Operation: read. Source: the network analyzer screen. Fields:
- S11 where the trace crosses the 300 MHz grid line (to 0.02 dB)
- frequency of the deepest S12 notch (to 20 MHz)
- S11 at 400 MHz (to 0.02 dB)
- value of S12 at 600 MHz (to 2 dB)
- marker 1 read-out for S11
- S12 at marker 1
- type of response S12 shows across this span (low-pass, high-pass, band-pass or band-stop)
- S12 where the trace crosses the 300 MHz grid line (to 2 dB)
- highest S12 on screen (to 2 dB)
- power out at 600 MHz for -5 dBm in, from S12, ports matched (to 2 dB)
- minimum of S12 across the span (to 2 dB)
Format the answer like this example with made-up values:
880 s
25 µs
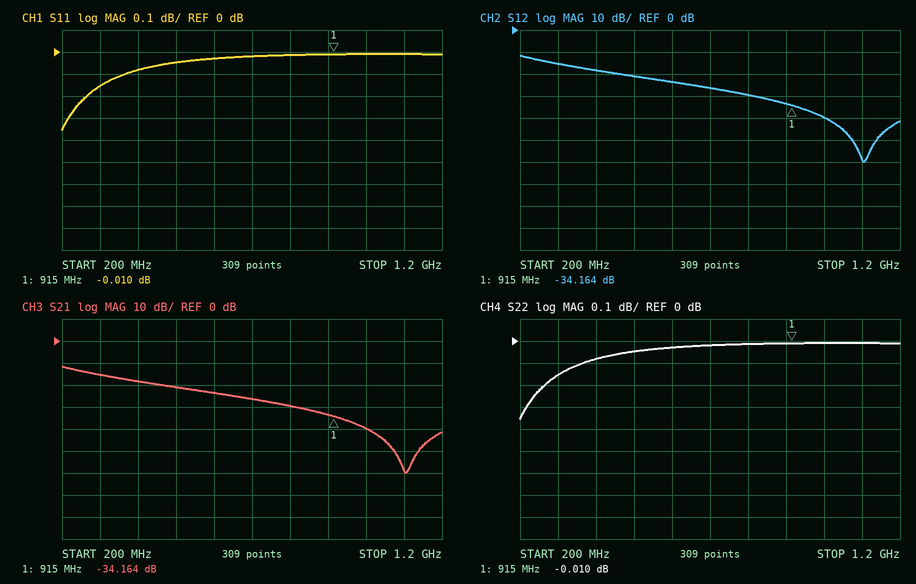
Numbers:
-0.16 dB
1.10 GHz
-0.08 dB
-24 dB
-0.010 dB
-34.164 dB
low-pass
-16 dB
-12 dB
-28 dBm
-60 dB
